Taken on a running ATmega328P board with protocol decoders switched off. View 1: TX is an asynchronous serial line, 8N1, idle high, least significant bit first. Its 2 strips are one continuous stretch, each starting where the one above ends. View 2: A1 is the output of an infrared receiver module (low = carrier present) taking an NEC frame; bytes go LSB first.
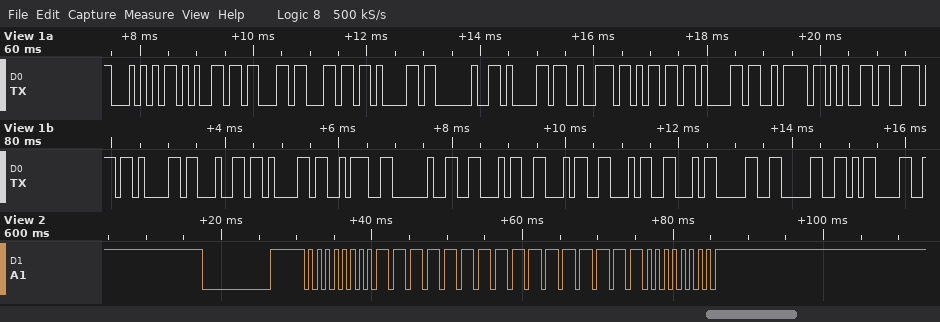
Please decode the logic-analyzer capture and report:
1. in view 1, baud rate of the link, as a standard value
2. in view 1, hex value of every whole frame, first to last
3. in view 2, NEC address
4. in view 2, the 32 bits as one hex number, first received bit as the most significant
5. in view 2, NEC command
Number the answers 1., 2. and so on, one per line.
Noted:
1. 9600 baud
2. 54 65 63 6C 61 20 61 72 6D 61 7A 65 6E 61 64 61 3A 20 46 46 46 46 30 30 0D
3. 0x00
4. 0x00FFFF00
5. 0xFF
